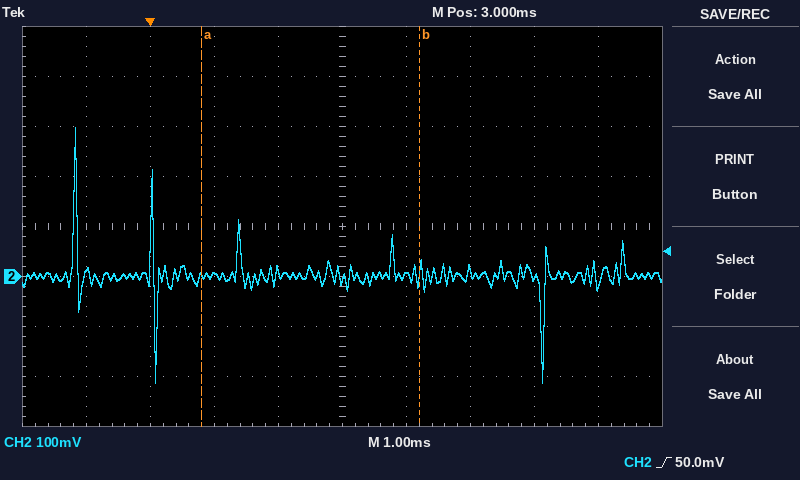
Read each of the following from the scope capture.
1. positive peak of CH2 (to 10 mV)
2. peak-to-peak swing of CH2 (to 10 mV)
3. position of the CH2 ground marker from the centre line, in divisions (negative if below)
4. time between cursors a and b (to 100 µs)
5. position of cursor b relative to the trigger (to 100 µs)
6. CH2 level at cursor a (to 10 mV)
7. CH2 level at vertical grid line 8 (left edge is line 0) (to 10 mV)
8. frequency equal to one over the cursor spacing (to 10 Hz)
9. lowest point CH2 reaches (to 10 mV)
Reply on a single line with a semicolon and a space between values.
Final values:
300 mV; 510 mV; -1.0 div; 3.4 ms; +4.2 ms; 0 mV; 0 mV; 290 Hz; -210 mV
